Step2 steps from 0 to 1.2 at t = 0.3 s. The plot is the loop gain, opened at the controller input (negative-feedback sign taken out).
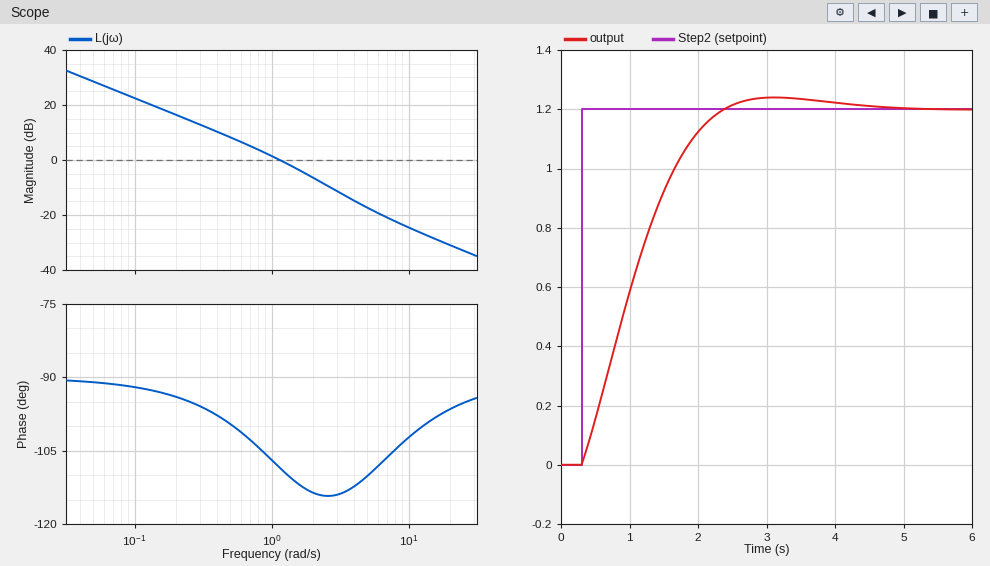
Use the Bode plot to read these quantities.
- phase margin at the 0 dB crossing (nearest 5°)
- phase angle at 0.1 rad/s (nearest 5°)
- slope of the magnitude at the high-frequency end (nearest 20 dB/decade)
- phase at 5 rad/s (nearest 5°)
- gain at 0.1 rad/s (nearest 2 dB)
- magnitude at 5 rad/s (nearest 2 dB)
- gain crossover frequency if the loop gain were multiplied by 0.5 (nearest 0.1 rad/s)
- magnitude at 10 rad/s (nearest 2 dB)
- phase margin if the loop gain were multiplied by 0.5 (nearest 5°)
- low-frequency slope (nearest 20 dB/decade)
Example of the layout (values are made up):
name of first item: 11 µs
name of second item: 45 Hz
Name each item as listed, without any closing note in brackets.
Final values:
phase margin at the 0 dB crossing: 70°
phase angle at 0.1 rad/s: -90°
slope of the magnitude at the high-frequency end: -20 dB/decade
phase at 5 rad/s: -110°
gain at 0.1 rad/s: 22 dB
magnitude at 5 rad/s: -18 dB
gain crossover frequency if the loop gain were multiplied by 0.5: 0.6 rad/s
magnitude at 10 rad/s: -24 dB
phase margin if the loop gain were multiplied by 0.5: 80°
low-frequency slope: -20 dB/decade
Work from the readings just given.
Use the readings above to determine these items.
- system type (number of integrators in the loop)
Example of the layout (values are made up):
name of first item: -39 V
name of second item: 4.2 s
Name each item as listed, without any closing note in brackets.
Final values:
system type: 1
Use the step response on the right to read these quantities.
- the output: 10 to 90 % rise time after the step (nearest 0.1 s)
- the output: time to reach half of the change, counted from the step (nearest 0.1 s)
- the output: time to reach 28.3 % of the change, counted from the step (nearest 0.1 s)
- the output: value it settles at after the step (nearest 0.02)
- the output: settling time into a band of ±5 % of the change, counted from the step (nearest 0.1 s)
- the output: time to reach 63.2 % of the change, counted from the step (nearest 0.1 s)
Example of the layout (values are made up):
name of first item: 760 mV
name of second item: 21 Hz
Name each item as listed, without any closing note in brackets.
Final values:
the output: 10 to 90 % rise time after the step: 1.4 s
the output: time to reach half of the change, counted from the step: 0.7 s
the output: time to reach 28.3 % of the change, counted from the step: 0.4 s
the output: value it settles at after the step: 1.20
the output: settling time into a band of ±5 % of the change, counted from the step: 1.8 s
the output: time to reach 63.2 % of the change, counted from the step: 0.9 s
